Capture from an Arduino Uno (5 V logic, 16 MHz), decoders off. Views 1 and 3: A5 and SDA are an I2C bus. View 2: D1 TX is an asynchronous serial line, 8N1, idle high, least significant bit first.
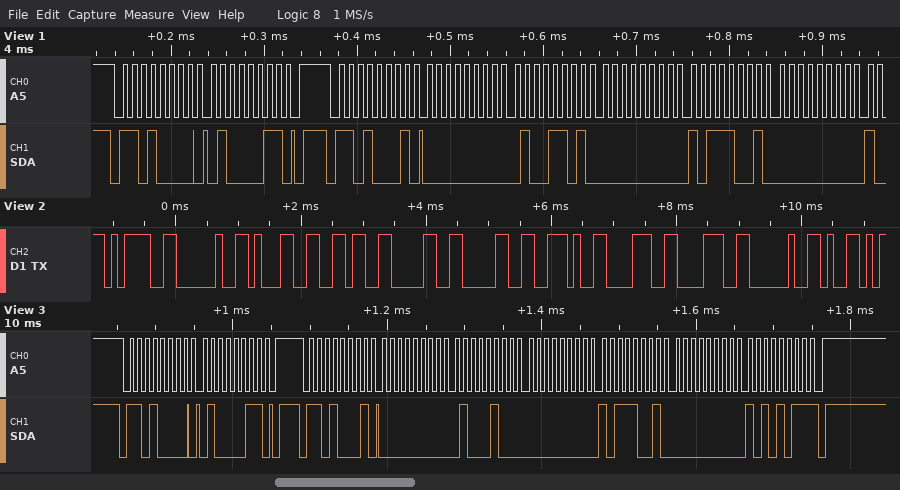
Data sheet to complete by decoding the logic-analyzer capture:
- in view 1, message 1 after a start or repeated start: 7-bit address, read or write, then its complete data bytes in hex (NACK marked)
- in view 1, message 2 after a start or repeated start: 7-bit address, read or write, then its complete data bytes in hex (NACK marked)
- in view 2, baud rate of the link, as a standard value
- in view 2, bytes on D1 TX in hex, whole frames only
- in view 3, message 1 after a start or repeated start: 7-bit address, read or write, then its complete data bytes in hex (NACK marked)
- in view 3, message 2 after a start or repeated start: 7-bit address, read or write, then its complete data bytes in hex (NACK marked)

0x68 write: 43
0x68 read: 00 4D 00 B9 00
9600 baud
3D 20 31 36 30 30 2E 38 38 20 59
0x68 write: 43
0x68 read: 00 44 00 B9 00 AB NACK
